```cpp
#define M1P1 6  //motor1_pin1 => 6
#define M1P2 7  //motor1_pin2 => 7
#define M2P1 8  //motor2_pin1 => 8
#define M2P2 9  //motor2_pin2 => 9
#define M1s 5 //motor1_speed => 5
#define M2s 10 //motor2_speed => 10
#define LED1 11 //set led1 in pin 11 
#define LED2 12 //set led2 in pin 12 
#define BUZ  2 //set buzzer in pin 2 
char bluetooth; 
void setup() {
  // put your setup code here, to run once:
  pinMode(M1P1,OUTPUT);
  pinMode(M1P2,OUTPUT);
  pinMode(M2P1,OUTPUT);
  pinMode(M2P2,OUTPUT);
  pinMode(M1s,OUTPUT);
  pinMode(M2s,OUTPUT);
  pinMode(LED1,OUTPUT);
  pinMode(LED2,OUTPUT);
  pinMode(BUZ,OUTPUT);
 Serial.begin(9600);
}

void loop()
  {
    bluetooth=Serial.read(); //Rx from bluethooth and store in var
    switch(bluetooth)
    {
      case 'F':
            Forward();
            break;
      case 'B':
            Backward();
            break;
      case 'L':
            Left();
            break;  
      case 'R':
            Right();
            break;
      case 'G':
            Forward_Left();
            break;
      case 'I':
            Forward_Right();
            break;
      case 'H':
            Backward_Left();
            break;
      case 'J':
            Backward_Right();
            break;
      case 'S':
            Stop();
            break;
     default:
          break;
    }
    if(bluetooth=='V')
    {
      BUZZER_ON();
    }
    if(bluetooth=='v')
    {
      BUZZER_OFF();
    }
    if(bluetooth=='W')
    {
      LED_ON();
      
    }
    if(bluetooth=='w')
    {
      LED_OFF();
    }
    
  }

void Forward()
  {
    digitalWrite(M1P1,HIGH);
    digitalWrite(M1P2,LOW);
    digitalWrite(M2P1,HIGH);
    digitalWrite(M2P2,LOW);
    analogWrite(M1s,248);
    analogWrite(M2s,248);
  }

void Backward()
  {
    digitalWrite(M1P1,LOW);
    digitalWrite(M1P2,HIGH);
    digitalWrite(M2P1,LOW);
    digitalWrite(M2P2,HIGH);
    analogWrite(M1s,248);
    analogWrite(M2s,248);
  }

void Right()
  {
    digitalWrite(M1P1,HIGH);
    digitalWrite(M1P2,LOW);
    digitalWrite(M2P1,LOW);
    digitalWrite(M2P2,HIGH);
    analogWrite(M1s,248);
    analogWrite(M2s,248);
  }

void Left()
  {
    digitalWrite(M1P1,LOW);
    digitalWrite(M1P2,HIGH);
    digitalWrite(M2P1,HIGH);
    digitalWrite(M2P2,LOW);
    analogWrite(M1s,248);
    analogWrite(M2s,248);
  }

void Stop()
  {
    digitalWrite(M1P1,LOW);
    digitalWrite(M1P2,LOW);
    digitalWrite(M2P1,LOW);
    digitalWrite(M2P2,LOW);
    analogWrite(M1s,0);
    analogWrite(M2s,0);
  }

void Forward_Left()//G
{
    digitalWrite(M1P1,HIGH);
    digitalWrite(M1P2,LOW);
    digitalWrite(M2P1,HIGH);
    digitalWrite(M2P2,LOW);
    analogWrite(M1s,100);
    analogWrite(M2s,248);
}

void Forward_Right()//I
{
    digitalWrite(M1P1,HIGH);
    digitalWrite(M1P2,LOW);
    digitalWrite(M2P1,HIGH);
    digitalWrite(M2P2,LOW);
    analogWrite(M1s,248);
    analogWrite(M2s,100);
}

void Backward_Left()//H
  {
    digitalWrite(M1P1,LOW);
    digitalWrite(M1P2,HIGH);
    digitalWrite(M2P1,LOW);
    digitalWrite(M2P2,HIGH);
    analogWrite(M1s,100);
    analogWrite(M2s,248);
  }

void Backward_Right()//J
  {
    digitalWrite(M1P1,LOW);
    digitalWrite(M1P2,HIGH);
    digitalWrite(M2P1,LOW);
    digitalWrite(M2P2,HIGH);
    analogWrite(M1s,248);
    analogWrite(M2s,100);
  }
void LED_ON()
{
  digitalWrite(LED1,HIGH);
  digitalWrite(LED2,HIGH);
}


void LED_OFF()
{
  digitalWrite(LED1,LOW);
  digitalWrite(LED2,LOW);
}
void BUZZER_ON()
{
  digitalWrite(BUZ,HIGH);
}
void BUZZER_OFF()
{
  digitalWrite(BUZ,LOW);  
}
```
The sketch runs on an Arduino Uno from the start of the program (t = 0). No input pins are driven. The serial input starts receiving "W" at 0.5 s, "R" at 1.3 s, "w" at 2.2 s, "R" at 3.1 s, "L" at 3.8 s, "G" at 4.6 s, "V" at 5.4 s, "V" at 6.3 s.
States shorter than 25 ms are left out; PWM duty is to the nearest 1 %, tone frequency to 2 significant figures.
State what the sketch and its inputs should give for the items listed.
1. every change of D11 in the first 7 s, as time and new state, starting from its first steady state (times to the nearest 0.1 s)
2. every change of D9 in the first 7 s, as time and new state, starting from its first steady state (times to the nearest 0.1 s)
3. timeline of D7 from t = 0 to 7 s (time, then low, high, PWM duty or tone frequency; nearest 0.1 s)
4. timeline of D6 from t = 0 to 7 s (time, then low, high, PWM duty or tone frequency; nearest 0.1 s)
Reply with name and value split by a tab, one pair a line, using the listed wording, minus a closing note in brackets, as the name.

every change of D11 in the first 7 s, as time and new state, starting from its first steady state	0 s low; 0.5 s high; 2.2 s low
every change of D9 in the first 7 s, as time and new state, starting from its first steady state	0 s low; 1.3 s high; 3.8 s low
timeline of D7 from t = 0 to 7 s	0 s low; 3.8 s high; 4.6 s low
timeline of D6 from t = 0 to 7 s	0 s low; 1.3 s high; 3.8 s low; 4.6 s high
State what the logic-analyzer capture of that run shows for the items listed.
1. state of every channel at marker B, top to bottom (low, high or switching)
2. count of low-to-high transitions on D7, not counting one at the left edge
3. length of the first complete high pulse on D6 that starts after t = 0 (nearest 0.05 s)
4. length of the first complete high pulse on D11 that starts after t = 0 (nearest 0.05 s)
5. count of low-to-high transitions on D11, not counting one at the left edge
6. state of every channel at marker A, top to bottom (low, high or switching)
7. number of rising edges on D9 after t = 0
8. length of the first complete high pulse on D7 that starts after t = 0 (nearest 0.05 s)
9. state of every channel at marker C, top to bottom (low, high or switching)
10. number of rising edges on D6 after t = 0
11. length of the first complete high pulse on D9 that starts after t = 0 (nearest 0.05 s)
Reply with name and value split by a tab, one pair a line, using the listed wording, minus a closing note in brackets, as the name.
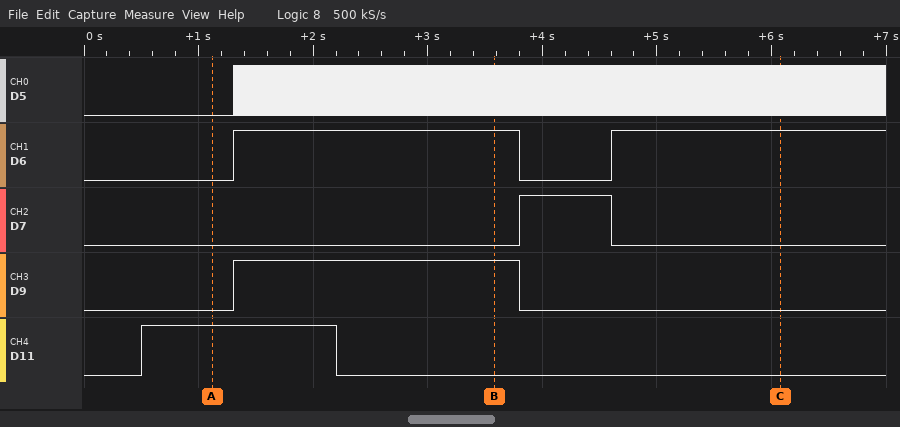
state of every channel at marker B, top to bottom	D5 switching, D6 high, D7 low, D9 high, D11 low
count of low-to-high transitions on D7, not counting one at the left edge	1
length of the first complete high pulse on D6 that starts after t = 0	2.50 s
length of the first complete high pulse on D11 that starts after t = 0	1.70 s
count of low-to-high transitions on D11, not counting one at the left edge	1
state of every channel at marker A, top to bottom	D5 low, D6 low, D7 low, D9 low, D11 high
number of rising edges on D9 after t = 0	1
length of the first complete high pulse on D7 that starts after t = 0	0.80 s
state of every channel at marker C, top to bottom	D5 switching, D6 high, D7 low, D9 low, D11 low
number of rising edges on D6 after t = 0	2
length of the first complete high pulse on D9 that starts after t = 0	2.50 s
